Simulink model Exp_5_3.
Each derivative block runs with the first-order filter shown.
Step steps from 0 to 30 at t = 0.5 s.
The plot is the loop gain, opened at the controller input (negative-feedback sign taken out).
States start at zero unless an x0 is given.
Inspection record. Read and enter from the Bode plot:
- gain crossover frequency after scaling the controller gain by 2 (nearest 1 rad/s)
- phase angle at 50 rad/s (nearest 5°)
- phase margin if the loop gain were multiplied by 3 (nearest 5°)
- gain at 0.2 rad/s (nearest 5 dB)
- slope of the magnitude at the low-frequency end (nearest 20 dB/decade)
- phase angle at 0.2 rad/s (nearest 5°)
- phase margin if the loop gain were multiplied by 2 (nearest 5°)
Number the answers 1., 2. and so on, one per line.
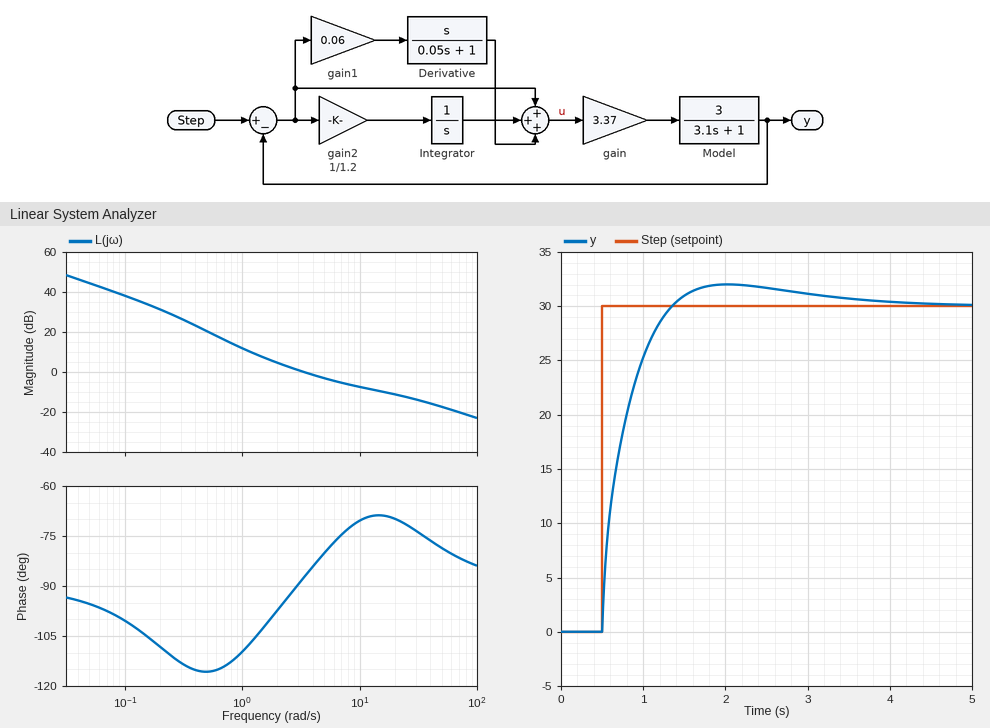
1. 8 rad/s
2. -80°
3. 110°
4. 30 dB
5. -20 dB/decade
6. -110°
7. 105°
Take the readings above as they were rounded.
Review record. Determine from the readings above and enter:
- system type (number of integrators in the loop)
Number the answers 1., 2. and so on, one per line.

1. 1
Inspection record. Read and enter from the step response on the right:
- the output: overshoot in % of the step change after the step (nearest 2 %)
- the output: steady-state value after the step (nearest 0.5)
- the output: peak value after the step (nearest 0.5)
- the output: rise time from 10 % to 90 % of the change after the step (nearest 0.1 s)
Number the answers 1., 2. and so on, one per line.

1. 6 %
2. 30.0
3. 32.0
4. 0.6 s
